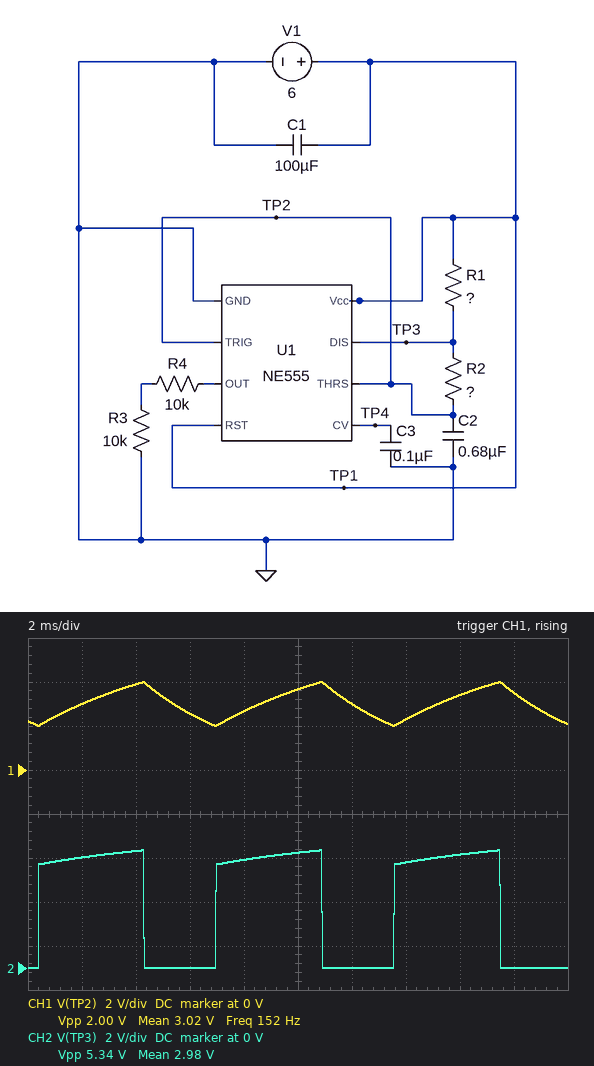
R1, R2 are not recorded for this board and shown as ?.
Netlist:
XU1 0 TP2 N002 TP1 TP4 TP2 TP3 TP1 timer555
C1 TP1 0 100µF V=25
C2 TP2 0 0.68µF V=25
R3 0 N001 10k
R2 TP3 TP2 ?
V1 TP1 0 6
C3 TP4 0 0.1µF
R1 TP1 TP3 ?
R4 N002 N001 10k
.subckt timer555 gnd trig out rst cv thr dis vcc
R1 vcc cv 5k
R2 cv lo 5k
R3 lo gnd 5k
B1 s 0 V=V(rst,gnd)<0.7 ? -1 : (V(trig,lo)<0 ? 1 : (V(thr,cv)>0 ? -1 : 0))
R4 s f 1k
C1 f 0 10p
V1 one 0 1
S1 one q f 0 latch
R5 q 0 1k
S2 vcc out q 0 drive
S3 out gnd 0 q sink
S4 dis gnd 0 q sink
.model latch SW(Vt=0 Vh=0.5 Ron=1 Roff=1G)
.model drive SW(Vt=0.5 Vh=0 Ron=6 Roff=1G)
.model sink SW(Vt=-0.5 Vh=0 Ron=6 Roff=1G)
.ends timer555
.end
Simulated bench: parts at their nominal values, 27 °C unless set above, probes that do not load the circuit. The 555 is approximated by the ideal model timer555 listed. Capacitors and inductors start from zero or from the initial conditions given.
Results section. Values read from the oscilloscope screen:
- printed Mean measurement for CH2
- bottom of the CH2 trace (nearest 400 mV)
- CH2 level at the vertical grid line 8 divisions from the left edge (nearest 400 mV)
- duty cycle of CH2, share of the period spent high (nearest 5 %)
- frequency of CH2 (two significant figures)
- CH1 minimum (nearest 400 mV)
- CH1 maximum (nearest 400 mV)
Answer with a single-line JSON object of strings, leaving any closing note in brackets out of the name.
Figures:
{"printed Mean measurement for CH2": "2.98 V", "bottom of the CH2 trace": "0 V", "CH2 level at the vertical grid line 8 divisions from the left edge": "5.2 V", "duty cycle of CH2, share of the period spent high": "60 %", "frequency of CH2": "150 Hz", "CH1 minimum": "2.0 V", "CH1 maximum": "4.0 V"}
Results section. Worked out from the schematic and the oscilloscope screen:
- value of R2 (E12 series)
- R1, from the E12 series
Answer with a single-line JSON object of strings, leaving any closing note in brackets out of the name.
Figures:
{"value of R2": "5.6 kΩ", "R1, from the E12 series": "2.7 kΩ"}
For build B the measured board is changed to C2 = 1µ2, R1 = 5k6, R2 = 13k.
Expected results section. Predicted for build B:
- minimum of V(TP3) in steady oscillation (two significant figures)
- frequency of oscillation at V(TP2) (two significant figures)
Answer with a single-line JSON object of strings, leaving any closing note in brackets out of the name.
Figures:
{"minimum of V(TP3) in steady oscillation": "7.3 mV", "frequency of oscillation at V(TP2)": "38 Hz"}
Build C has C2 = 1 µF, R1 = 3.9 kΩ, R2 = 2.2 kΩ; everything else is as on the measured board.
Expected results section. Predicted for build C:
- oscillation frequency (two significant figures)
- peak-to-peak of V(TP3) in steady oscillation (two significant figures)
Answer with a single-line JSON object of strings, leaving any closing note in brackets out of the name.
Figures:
{"oscillation frequency": "170 Hz", "peak-to-peak of V(TP3) in steady oscillation": "4.7 V"}
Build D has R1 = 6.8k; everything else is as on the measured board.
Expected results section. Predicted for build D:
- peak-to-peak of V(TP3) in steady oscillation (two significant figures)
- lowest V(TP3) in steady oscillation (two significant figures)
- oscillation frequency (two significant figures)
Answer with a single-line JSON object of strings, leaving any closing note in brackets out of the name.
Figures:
{"peak-to-peak of V(TP3) in steady oscillation": "4.9 V", "lowest V(TP3) in steady oscillation": "7.4 mV", "oscillation frequency": "120 Hz"}
